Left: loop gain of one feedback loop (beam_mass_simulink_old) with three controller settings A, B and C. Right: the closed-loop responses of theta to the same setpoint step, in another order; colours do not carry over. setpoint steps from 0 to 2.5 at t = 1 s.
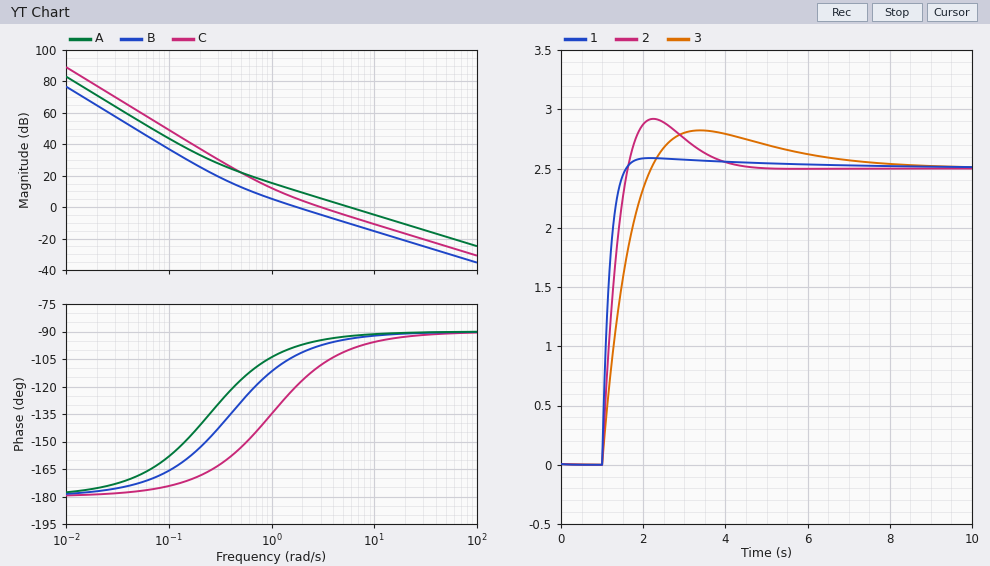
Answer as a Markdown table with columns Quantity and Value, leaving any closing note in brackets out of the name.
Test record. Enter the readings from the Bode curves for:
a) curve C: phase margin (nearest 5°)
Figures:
| Quantity | Value |
|---|---|
| curve C: phase margin | 70° |
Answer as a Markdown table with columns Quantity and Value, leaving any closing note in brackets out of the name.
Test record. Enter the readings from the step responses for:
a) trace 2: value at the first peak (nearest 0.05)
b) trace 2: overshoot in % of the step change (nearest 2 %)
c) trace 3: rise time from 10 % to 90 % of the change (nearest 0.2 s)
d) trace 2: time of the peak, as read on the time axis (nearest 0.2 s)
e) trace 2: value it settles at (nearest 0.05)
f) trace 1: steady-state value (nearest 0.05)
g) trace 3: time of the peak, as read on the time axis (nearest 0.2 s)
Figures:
| Quantity | Value |
|---|---|
| trace 2: value at the first peak | 2.90 |
| trace 2: overshoot in % of the step change | 16 % |
| trace 3: rise time from 10 % to 90 % of the change | 0.8 s |
| trace 2: time of the peak, as read on the time axis | 2.2 s |
| trace 2: value it settles at | 2.50 |
| trace 1: steady-state value | 2.50 |
| trace 3: time of the peak, as read on the time axis | 3.4 s |
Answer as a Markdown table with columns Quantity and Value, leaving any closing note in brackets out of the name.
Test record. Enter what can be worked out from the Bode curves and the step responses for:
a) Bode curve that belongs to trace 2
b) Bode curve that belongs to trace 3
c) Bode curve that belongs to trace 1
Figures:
| Quantity | Value |
|---|---|
| Bode curve that belongs to trace 2 | C |
| Bode curve that belongs to trace 3 | B |
| Bode curve that belongs to trace 1 | A |
